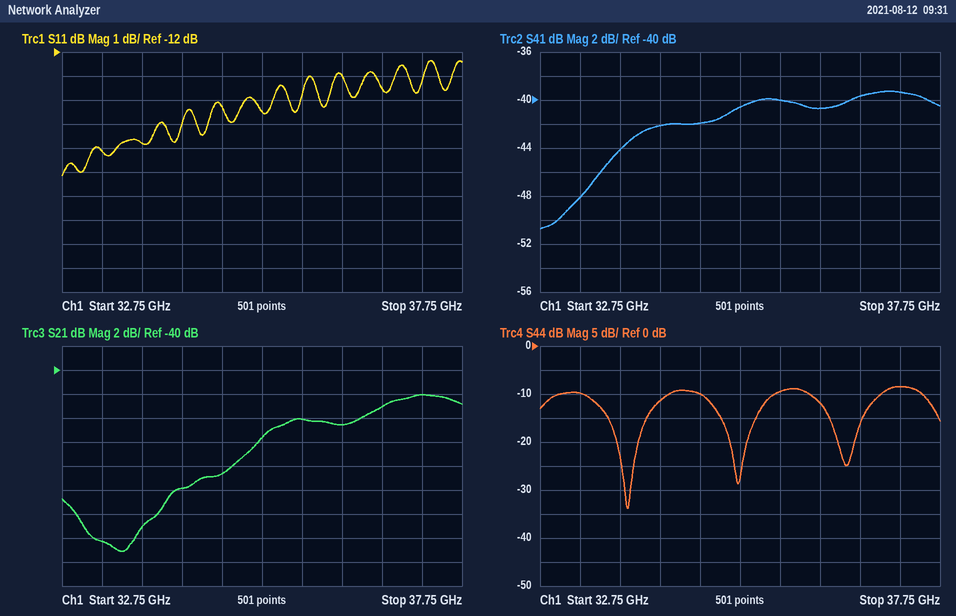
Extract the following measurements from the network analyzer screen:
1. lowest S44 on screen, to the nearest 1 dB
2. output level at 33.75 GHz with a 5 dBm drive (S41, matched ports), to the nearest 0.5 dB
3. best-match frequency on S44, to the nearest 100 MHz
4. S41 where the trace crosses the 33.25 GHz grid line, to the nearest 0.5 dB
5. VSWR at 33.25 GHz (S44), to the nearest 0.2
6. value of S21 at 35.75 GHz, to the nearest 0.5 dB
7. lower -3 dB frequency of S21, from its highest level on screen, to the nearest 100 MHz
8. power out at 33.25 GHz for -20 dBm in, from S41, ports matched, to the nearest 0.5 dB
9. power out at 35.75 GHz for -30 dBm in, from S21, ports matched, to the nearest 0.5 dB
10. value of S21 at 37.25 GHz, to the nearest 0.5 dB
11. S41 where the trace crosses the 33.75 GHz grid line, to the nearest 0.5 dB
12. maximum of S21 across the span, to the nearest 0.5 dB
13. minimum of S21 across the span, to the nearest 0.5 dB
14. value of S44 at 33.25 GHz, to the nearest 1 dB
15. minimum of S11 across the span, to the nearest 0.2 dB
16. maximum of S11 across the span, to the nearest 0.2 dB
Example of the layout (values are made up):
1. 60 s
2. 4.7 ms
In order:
1. -34 dB
2. -39.0 dBm
3. 33.8 GHz
4. -48.0 dB
5. 2.0
6. -44.0 dB
7. 35.3 GHz
8. -68.0 dBm
9. -74.0 dBm
10. -42.0 dB
11. -44.0 dB
12. -42.0 dB
13. -55.0 dB
14. -10 dB
15. -17.2 dB
16. -12.4 dB
